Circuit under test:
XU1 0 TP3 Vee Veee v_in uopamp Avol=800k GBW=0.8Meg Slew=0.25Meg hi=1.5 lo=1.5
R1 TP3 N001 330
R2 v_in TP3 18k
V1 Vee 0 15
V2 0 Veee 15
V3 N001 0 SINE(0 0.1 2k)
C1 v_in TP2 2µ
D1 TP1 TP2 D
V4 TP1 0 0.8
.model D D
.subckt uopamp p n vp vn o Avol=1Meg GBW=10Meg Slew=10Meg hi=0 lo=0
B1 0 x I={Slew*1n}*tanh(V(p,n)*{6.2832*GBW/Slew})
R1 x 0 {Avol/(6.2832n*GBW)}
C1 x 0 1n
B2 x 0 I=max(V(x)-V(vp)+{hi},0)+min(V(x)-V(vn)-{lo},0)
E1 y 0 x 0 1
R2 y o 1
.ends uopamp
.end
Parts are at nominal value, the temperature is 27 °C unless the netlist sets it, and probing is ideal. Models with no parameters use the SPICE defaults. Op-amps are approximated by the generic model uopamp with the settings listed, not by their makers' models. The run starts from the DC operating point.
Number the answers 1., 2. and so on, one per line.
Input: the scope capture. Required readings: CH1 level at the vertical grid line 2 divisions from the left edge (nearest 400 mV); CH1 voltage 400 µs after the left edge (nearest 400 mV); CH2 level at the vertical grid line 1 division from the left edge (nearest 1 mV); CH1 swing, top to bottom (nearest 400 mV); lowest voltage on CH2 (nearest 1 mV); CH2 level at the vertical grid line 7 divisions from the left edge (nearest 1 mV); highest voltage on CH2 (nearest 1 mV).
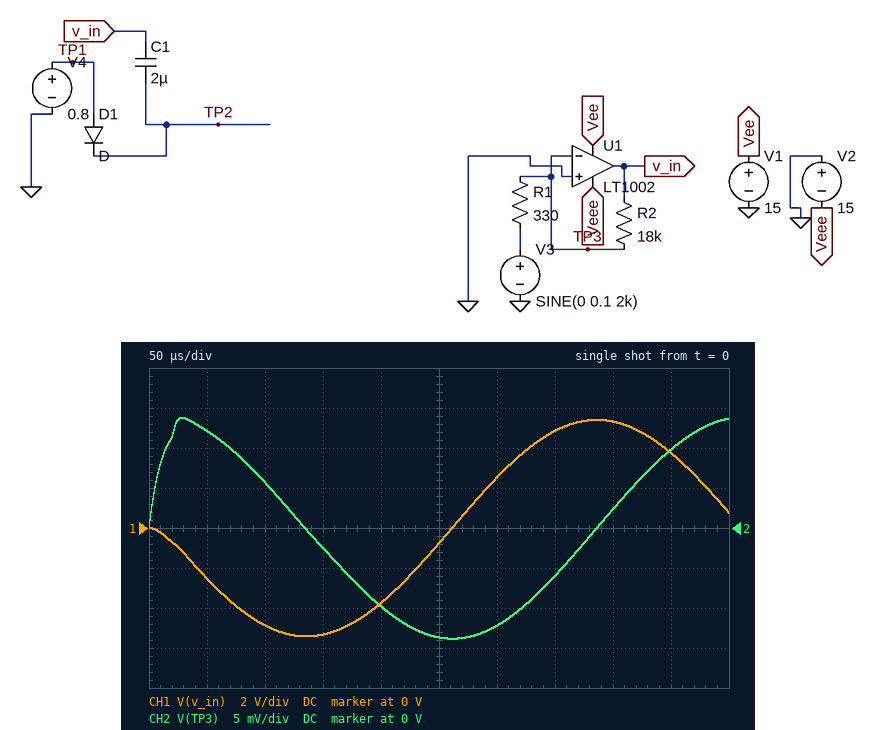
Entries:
1. -4.8 V
2. 5.2 V
3. 12 mV
4. 10.8 V
5. -14 mV
6. -6 mV
7. 14 mV
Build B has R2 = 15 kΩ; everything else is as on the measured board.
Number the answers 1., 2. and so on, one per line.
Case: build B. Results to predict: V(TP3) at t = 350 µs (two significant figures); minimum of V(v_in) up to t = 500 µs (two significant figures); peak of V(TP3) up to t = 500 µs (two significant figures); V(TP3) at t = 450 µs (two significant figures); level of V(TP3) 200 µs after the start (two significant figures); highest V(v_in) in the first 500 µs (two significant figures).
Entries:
1. -4.7 mV
2. -4.5 V
3. 12 mV
4. 8.4 mV
5. -8.4 mV
6. 4.5 V
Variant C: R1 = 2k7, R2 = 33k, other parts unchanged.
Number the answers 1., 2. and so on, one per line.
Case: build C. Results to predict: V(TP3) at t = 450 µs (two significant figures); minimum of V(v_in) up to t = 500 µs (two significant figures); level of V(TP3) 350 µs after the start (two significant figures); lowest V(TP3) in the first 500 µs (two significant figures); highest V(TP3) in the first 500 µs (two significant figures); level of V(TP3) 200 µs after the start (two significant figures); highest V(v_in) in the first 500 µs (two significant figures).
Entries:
1. 2.4 mV
2. -1.2 V
3. -1.0 mV
4. -3.1 mV
5. 3.1 mV
6. -2.4 mV
7. 1.2 V
